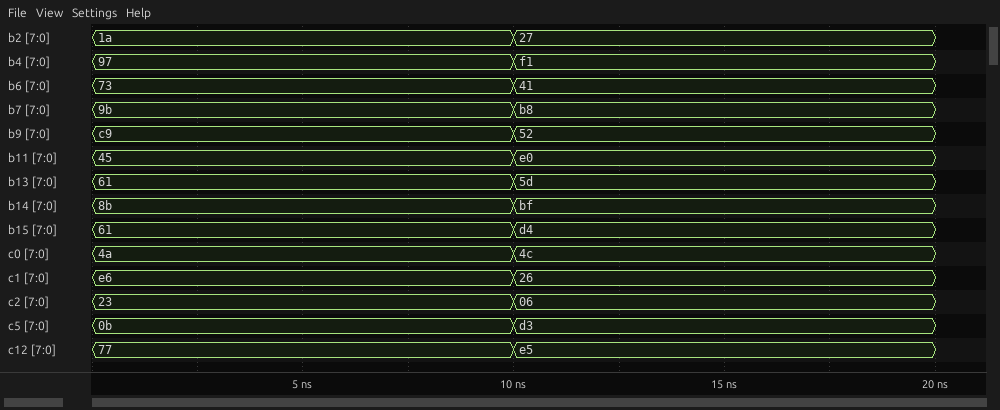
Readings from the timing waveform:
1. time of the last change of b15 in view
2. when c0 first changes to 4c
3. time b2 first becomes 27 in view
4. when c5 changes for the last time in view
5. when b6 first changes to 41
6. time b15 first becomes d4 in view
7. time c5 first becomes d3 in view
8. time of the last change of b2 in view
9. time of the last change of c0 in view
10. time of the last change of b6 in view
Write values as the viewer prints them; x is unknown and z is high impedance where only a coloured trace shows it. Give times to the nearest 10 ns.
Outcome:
10 ns
10 ns
10 ns
10 ns
10 ns
10 ns
10 ns
10 ns
10 ns
10 ns
